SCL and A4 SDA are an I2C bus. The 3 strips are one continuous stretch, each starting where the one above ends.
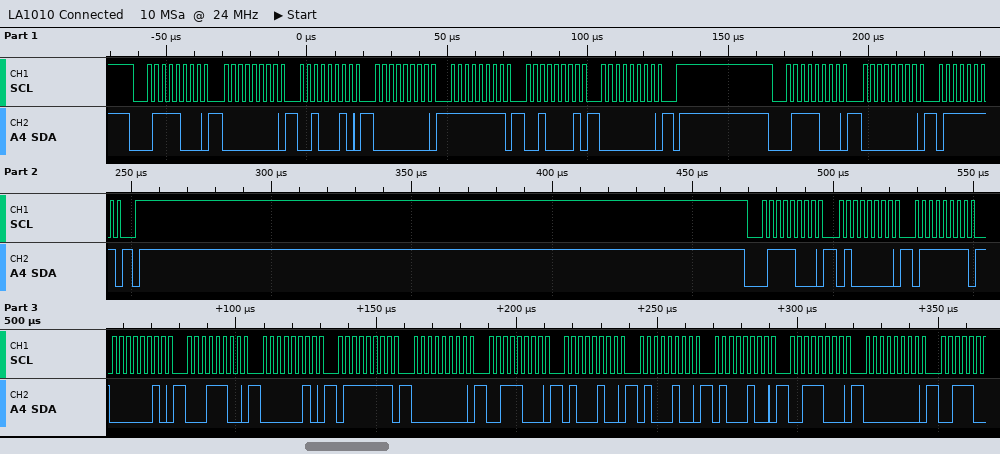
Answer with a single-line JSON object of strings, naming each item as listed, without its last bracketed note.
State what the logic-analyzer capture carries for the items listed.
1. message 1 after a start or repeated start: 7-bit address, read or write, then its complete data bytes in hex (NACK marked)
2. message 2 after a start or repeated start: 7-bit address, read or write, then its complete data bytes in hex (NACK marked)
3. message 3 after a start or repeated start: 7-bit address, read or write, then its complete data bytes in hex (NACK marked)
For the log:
{"message 1 after a start or repeated start: 7-bit address, read or write, then its complete data bytes in hex": "0x3C write: 00 22 00 FF 21 00", "message 2 after a start or repeated start: 7-bit address, read or write, then its complete data bytes in hex": "0x3C write: 00 7F", "message 3 after a start or repeated start: 7-bit address, read or write, then its complete data bytes in hex": "0x3C write: 40 7F 02 1C 02 7F 00 38 44 44 44 38 00"}
